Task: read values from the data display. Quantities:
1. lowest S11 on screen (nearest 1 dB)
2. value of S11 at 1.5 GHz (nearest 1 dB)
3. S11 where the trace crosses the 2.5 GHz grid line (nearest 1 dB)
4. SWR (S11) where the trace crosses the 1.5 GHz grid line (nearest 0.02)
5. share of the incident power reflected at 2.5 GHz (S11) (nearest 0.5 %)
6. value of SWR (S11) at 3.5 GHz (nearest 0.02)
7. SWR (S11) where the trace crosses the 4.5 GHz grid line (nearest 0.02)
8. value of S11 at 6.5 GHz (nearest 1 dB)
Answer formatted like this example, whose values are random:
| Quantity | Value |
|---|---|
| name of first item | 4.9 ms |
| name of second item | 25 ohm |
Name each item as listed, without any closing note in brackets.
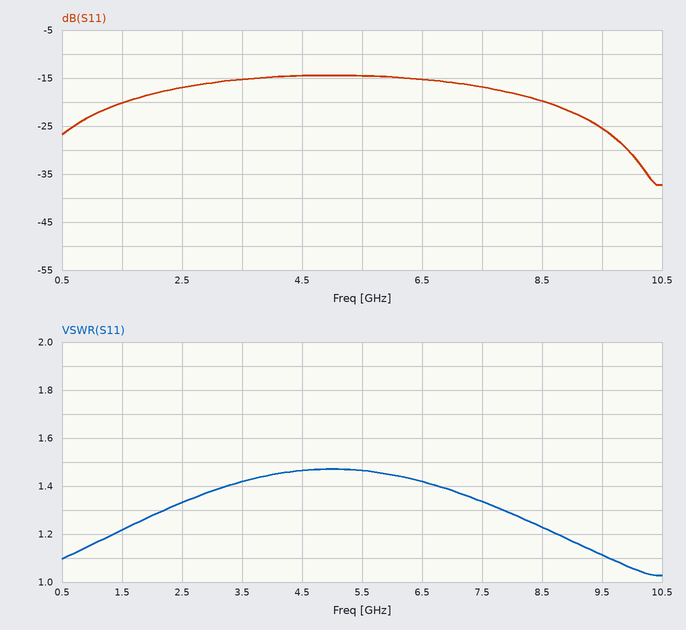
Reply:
| Quantity | Value |
|---|---|
| lowest S11 on screen | -37 dB |
| value of S11 at 1.5 GHz | -20 dB |
| S11 where the trace crosses the 2.5 GHz grid line | -17 dB |
| SWR (S11) where the trace crosses the 1.5 GHz grid line | 1.22 |
| share of the incident power reflected at 2.5 GHz (S11) | 2.0 % |
| value of SWR (S11) at 3.5 GHz | 1.42 |
| SWR (S11) where the trace crosses the 4.5 GHz grid line | 1.46 |
| value of S11 at 6.5 GHz | -15 dB |
